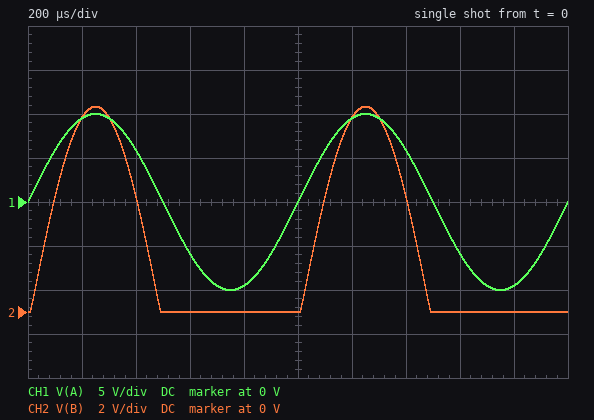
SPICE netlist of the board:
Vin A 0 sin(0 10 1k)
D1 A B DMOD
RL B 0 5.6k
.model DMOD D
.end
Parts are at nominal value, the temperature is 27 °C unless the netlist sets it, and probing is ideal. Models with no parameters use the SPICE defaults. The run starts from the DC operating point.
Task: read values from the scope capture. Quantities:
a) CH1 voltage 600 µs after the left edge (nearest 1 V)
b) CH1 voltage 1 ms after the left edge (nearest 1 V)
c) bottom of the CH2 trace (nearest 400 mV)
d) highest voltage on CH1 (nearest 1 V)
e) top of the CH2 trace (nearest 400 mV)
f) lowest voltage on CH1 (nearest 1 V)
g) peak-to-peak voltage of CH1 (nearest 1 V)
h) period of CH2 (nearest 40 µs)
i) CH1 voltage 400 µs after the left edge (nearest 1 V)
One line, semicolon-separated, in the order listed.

-6 V; 0 V; 0 V; 10 V; 9.2 V; -10 V; 20 V; 1.00 ms; 6 V
